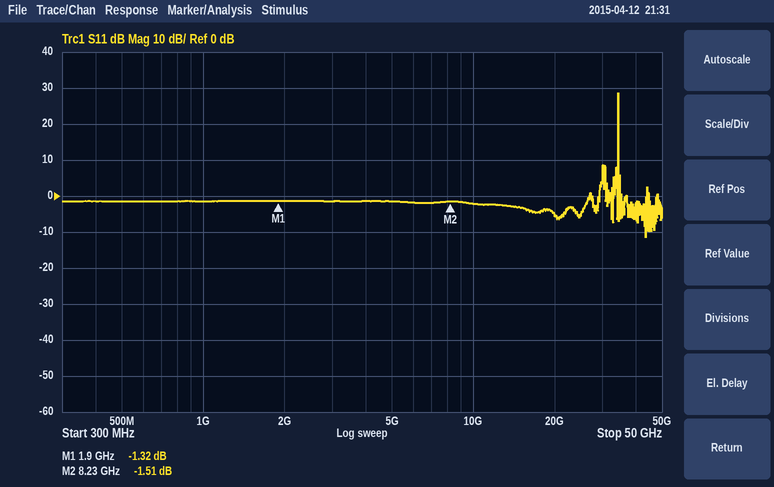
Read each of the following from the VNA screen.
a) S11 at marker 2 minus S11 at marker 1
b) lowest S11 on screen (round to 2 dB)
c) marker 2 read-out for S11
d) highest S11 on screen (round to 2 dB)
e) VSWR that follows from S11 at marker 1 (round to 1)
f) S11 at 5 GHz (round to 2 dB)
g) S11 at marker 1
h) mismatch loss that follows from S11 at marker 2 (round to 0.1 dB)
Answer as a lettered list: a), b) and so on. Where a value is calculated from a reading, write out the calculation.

a) -1.51 − (-1.32) = -0.19 dB
b) -12 dB
c) -1.51 dB
d) 28 dB
e) (1 + 0.8590)/(1 − 0.8590) ≈ 13
f) -2 dB
g) -1.32 dB
h) −10 log10(1 − 10^(-1.51/10)) ≈ 5.3 dB
